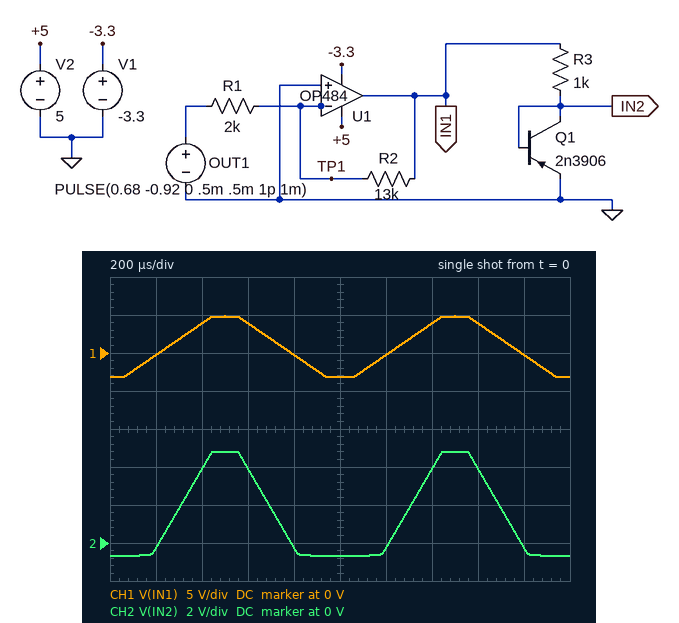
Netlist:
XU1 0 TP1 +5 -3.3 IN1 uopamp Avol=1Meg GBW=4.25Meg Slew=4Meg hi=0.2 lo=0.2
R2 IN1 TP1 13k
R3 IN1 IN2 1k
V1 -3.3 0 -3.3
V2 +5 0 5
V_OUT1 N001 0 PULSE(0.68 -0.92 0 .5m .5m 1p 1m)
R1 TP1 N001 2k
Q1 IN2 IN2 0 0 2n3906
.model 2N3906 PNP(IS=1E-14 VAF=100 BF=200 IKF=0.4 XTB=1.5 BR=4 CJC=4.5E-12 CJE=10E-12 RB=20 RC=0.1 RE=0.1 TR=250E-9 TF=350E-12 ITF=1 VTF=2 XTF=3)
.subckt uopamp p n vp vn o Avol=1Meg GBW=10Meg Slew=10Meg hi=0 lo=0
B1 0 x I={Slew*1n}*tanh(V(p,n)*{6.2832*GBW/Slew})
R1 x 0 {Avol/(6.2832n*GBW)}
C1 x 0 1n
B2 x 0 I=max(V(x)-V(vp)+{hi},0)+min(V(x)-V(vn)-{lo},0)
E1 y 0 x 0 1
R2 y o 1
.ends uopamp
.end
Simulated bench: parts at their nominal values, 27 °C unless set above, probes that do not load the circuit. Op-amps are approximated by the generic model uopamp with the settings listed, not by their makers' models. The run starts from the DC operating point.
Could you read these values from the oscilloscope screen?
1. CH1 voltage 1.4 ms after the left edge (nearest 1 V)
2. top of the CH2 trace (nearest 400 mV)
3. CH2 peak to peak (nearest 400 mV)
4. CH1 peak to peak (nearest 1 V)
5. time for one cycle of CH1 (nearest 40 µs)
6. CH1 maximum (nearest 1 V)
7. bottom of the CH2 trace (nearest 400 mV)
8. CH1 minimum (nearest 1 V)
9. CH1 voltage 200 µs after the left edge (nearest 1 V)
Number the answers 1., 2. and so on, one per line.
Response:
1. 4 V
2. 4.8 V
3. 5.6 V
4. 8 V
5. 1.00 ms
6. 5 V
7. -800 mV
8. -3 V
9. 0 V
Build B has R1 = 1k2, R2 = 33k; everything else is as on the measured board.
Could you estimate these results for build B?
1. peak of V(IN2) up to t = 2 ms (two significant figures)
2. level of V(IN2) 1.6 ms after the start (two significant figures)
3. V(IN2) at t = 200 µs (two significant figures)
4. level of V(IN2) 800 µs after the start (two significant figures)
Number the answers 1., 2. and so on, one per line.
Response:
1. 4.8 V
2. 4.8 V
3. -640 mV
4. -630 mV
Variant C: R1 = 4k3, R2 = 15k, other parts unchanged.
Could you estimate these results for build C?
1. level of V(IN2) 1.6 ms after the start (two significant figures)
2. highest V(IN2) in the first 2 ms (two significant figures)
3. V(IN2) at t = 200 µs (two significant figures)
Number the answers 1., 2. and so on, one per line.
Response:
1. 2.1 V
2. 3.2 V
3. -140 mV
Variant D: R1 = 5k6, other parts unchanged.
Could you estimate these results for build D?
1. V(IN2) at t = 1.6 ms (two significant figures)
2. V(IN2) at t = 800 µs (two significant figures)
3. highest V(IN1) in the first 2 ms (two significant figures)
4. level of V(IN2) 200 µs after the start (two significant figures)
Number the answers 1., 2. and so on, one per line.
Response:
1. 1.4 V
2. -92 mV
3. 2.1 V
4. -94 mV
